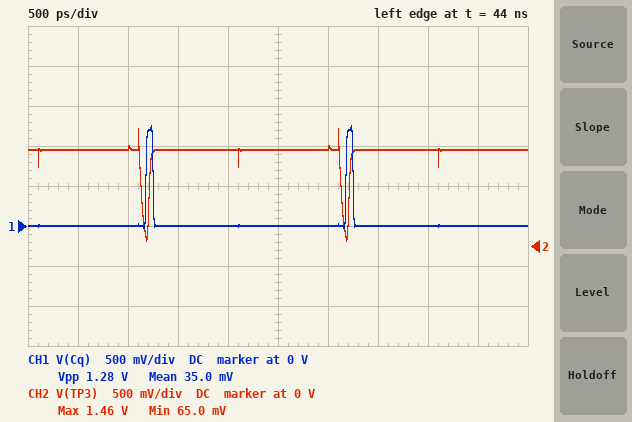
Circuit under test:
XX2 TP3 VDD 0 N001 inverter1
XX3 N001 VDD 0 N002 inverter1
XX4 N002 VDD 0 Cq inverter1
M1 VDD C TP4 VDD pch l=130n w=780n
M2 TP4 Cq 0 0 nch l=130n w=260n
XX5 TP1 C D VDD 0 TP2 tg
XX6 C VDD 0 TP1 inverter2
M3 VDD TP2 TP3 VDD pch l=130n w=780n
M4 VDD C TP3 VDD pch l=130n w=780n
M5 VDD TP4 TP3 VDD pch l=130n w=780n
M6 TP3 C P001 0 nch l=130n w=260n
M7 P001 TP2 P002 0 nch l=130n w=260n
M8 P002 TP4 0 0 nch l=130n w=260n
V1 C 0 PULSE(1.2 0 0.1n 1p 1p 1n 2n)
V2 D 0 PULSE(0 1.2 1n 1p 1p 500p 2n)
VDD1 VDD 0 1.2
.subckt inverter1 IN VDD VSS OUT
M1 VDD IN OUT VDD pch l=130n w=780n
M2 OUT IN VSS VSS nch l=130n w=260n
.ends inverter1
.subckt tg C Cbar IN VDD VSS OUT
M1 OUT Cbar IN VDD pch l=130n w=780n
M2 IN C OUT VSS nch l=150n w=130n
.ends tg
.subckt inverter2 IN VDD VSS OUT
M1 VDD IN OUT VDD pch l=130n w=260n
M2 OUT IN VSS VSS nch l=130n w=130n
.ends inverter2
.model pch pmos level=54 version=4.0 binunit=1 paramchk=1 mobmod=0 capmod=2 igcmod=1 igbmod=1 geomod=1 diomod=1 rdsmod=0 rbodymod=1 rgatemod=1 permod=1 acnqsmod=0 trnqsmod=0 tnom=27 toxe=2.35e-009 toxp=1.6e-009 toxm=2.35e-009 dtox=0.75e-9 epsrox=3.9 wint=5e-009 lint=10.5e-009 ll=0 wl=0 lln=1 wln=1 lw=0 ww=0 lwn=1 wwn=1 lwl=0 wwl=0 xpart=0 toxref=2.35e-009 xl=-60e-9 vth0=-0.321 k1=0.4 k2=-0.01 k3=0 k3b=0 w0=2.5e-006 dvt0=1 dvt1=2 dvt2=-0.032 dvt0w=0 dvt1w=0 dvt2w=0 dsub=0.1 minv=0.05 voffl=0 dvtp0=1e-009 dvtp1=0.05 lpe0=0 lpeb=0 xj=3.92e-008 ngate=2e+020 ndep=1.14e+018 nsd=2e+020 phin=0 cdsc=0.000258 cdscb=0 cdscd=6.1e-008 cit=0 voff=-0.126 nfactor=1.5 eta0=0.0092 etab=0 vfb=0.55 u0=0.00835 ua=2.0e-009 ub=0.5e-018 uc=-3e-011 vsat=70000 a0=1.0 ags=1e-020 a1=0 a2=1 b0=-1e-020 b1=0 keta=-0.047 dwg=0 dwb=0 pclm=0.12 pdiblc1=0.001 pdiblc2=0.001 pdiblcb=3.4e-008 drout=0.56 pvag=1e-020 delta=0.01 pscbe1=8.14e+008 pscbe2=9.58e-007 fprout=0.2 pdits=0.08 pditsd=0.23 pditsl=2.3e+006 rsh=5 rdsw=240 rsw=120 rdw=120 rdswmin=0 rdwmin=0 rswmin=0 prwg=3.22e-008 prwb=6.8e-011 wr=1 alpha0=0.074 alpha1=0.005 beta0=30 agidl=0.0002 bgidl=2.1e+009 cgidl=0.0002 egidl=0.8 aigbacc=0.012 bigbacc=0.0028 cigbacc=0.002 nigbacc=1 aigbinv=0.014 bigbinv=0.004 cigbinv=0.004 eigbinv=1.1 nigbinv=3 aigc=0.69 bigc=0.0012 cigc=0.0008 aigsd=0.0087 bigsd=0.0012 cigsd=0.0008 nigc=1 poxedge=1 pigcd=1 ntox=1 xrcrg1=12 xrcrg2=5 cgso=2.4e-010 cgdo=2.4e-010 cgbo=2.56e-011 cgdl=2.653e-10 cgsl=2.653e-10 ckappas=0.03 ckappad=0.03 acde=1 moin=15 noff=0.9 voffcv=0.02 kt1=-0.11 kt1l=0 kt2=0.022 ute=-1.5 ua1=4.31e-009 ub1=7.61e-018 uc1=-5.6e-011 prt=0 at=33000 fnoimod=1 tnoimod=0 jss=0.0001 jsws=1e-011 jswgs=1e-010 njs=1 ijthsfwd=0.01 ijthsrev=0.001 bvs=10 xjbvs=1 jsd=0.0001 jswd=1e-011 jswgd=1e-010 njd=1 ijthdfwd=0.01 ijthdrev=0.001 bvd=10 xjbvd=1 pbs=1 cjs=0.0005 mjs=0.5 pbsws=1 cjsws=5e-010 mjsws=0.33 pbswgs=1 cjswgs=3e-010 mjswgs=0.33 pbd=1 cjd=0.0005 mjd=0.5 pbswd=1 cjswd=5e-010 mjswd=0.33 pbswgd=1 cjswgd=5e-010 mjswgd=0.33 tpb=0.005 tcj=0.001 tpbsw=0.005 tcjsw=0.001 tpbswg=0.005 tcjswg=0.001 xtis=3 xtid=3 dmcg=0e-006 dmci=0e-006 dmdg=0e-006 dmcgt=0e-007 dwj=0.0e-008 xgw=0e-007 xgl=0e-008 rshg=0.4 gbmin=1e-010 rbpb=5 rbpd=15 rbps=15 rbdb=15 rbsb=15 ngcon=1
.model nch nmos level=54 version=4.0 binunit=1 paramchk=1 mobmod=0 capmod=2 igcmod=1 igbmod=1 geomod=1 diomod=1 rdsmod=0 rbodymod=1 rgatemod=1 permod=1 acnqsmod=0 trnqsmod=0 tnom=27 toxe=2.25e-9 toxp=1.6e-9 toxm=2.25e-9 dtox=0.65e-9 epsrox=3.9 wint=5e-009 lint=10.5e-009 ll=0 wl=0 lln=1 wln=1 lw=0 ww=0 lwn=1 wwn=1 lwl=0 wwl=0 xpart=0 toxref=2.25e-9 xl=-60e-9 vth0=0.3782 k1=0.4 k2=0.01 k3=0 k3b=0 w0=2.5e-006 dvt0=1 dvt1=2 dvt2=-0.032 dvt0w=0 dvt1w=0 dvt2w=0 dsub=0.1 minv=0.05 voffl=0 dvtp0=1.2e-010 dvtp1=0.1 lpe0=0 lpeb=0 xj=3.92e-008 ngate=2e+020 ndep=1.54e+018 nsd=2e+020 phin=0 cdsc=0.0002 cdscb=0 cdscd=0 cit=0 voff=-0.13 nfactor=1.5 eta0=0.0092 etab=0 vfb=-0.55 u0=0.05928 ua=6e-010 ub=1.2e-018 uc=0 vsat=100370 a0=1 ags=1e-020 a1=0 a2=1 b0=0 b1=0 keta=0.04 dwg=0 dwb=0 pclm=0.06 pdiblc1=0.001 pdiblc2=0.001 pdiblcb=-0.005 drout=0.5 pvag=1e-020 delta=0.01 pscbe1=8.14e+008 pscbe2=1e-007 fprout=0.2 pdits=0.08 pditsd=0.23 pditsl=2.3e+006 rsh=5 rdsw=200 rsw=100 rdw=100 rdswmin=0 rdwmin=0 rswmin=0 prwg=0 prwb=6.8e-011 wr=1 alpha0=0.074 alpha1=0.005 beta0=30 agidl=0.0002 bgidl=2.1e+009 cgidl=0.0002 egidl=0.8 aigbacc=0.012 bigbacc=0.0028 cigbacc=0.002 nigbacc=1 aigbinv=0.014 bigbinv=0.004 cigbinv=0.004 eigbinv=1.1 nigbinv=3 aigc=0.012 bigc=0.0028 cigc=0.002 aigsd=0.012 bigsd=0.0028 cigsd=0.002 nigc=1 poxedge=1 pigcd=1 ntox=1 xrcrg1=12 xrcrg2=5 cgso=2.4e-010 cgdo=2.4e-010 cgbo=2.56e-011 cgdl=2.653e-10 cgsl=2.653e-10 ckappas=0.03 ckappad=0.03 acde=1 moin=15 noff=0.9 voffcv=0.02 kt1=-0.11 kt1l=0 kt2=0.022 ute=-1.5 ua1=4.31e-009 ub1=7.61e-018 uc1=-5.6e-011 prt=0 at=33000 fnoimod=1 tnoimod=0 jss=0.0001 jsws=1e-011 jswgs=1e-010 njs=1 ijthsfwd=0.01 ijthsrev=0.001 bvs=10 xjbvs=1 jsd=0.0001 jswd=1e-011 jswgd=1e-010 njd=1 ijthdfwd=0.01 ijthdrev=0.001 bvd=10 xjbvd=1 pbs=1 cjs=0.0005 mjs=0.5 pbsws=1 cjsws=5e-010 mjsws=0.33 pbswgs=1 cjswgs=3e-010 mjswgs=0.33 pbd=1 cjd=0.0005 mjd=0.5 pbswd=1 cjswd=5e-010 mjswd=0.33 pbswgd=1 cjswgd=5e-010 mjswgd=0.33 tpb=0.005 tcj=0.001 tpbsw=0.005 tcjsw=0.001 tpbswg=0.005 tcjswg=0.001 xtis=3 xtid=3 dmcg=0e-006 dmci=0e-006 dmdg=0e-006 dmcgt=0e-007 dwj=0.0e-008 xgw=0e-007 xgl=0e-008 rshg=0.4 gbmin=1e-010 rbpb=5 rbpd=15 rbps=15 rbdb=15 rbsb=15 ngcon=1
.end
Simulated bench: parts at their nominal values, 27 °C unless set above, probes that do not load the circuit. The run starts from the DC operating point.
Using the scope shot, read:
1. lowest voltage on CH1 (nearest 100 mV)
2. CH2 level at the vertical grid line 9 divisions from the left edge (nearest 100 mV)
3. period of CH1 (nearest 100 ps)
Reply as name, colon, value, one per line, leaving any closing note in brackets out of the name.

lowest voltage on CH1: 0 V
CH2 level at the vertical grid line 9 divisions from the left edge: 1.2 V
period of CH1: 2.0 ns
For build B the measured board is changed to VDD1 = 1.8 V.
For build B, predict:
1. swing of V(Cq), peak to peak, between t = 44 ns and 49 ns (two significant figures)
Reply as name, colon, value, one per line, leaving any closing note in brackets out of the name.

swing of V(Cq), peak to peak, between t = 44 ns and 49 ns: 1.6 V
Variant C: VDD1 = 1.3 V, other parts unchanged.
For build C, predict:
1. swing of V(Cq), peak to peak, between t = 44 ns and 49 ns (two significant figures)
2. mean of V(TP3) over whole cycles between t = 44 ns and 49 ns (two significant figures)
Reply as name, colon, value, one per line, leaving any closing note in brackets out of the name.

swing of V(Cq), peak to peak, between t = 44 ns and 49 ns: 1.4 V
mean of V(TP3) over whole cycles between t = 44 ns and 49 ns: 1.3 V
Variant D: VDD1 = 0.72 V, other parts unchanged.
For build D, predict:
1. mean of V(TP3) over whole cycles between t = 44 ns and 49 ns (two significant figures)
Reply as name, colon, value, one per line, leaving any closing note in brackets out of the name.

mean of V(TP3) over whole cycles between t = 44 ns and 49 ns: 670 mV
